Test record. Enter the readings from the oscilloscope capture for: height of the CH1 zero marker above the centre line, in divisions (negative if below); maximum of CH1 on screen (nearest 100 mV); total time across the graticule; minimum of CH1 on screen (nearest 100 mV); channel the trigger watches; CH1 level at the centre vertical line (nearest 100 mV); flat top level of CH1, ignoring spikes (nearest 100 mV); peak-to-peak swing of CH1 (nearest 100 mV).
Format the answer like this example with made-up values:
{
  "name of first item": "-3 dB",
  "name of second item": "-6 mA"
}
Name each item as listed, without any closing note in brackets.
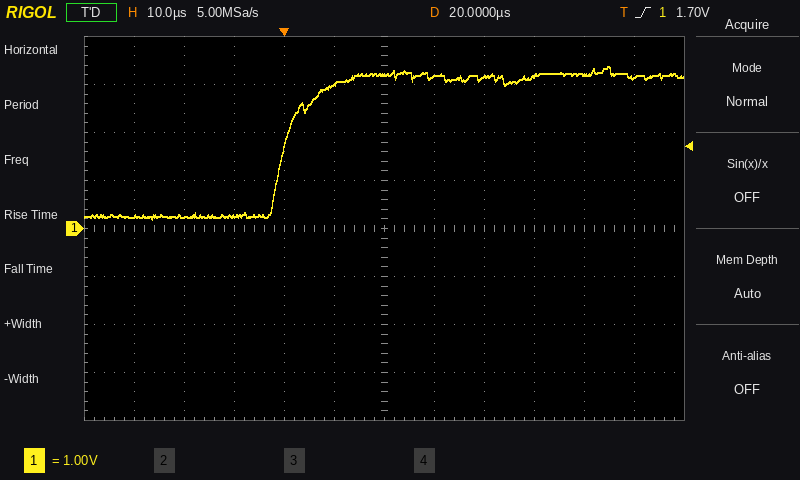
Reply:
{
  "height of the CH1 zero marker above the centre line, in divisions": "0.0 div",
  "maximum of CH1 on screen": "3.4 V",
  "total time across the graticule": "120 µs",
  "minimum of CH1 on screen": "200 mV",
  "channel the trigger watches": "CH1",
  "CH1 level at the centre vertical line": "3.2 V",
  "flat top level of CH1, ignoring spikes": "3.2 V",
  "peak-to-peak swing of CH1": "3.2 V"
}
